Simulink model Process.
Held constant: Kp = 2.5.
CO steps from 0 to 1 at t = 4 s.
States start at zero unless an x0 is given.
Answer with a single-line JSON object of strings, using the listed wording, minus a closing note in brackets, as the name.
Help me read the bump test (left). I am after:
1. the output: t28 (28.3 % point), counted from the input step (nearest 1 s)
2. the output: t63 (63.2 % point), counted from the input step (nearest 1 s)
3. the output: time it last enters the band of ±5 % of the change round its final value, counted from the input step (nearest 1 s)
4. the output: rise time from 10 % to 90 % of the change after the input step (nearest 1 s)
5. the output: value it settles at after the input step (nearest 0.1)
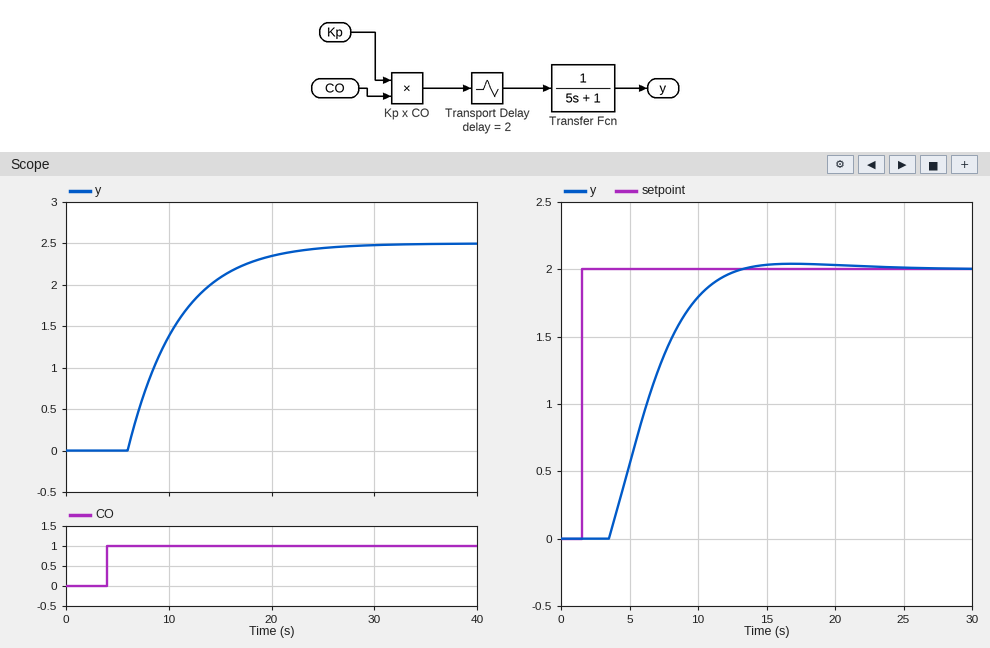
{"the output: t28 (28.3 % point), counted from the input step": "4 s", "the output: t63 (63.2 % point), counted from the input step": "7 s", "the output: time it last enters the band of ±5 % of the change round its final value, counted from the input step": "17 s", "the output: rise time from 10 % to 90 % of the change after the input step": "11 s", "the output: value it settles at after the input step": "2.5"}
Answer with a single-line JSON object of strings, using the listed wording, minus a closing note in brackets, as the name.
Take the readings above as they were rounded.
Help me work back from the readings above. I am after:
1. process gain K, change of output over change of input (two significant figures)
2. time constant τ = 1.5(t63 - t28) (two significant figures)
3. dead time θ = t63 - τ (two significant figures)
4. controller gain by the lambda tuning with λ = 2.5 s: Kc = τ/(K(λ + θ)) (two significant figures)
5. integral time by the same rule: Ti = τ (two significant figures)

{"process gain K, change of output over change of input": "2.5", "time constant τ = 1.5(t63 - t28)": "4.5 s", "dead time θ = t63 - τ": "2.5 s", "controller gain by the lambda tuning with λ = 2.5 s: Kc = τ/(K(λ + θ))": "0.36", "integral time by the same rule: Ti = τ": "4.5 s"}
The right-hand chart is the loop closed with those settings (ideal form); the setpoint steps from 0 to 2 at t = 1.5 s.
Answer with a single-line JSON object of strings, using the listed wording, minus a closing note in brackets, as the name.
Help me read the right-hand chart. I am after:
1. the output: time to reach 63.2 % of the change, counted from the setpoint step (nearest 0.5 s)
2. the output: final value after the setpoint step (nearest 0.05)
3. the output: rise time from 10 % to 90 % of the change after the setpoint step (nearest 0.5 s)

{"the output: time to reach 63.2 % of the change, counted from the setpoint step": "5.5 s", "the output: final value after the setpoint step": "2.00", "the output: rise time from 10 % to 90 % of the change after the setpoint step": "6.0 s"}
